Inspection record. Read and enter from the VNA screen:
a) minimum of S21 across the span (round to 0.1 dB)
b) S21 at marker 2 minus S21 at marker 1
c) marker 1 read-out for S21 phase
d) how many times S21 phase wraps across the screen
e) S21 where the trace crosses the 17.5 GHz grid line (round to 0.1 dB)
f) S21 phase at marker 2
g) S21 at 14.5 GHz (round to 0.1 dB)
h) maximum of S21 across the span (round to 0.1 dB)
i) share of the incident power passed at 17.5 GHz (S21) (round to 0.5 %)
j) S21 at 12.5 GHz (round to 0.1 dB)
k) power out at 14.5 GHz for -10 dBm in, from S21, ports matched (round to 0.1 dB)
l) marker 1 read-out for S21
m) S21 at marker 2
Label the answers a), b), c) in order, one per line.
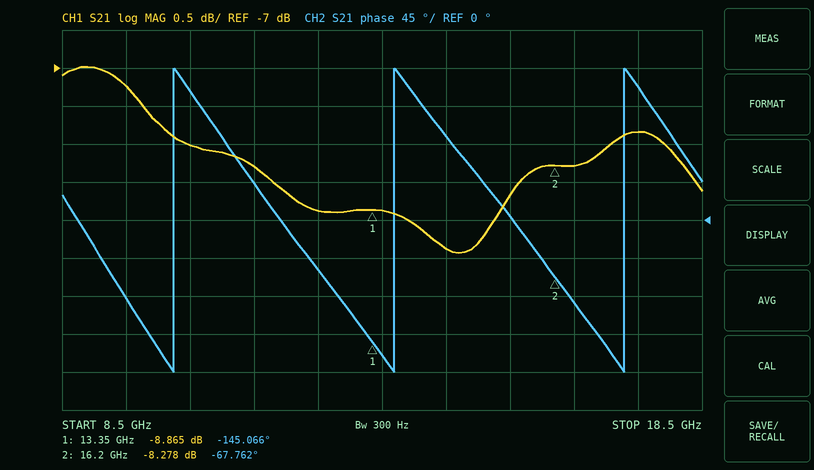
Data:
a) -9.4 dB
b) 0.587 dB
c) -145.066°
d) 3
e) -7.8 dB
f) -67.762°
g) -9.4 dB
h) -7.0 dB
i) 16.5 %
j) -8.9 dB
k) -19.4 dBm
l) -8.865 dB
m) -8.278 dB
